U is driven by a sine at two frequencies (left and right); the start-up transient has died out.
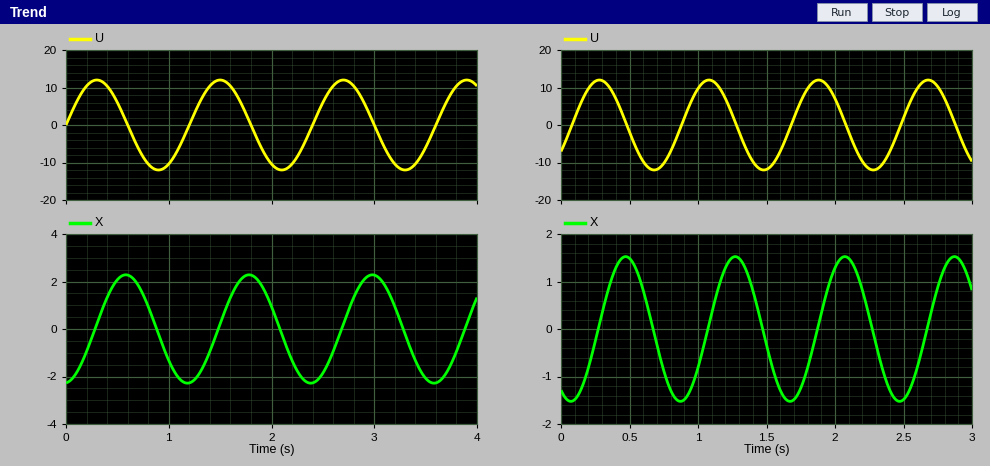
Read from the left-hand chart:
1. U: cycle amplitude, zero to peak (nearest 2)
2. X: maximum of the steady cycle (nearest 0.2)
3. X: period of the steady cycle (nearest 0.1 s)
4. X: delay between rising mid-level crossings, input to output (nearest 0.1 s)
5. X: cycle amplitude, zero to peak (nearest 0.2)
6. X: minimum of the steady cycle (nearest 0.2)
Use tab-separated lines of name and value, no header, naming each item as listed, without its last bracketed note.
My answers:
U: cycle amplitude, zero to peak	12
X: maximum of the steady cycle	2.2
X: period of the steady cycle	1.2 s
X: delay between rising mid-level crossings, input to output	0.3 s
X: cycle amplitude, zero to peak	2.2
X: minimum of the steady cycle	-2.2
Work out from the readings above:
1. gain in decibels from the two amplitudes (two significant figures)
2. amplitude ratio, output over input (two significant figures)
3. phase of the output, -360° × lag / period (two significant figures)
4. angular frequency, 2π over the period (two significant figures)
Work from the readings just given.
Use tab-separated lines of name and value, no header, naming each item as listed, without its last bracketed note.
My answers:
gain in decibels from the two amplitudes	-15 dB
amplitude ratio, output over input	0.18
phase of the output, -360° × lag / period	-90°
angular frequency, 2π over the period	5.2 rad/s
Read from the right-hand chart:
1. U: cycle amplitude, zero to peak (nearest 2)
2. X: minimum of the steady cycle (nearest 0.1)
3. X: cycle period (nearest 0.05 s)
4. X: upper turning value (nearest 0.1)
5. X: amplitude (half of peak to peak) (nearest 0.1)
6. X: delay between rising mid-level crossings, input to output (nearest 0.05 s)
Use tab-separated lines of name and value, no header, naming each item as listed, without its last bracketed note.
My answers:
U: cycle amplitude, zero to peak	12
X: minimum of the steady cycle	-1.5
X: cycle period	0.80 s
X: upper turning value	1.5
X: amplitude (half of peak to peak)	1.5
X: delay between rising mid-level crossings, input to output	0.20 s
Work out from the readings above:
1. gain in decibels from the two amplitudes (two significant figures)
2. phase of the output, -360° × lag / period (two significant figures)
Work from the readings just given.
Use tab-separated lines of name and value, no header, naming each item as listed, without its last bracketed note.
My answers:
gain in decibels from the two amplitudes	-18 dB
phase of the output, -360° × lag / period	-90°
